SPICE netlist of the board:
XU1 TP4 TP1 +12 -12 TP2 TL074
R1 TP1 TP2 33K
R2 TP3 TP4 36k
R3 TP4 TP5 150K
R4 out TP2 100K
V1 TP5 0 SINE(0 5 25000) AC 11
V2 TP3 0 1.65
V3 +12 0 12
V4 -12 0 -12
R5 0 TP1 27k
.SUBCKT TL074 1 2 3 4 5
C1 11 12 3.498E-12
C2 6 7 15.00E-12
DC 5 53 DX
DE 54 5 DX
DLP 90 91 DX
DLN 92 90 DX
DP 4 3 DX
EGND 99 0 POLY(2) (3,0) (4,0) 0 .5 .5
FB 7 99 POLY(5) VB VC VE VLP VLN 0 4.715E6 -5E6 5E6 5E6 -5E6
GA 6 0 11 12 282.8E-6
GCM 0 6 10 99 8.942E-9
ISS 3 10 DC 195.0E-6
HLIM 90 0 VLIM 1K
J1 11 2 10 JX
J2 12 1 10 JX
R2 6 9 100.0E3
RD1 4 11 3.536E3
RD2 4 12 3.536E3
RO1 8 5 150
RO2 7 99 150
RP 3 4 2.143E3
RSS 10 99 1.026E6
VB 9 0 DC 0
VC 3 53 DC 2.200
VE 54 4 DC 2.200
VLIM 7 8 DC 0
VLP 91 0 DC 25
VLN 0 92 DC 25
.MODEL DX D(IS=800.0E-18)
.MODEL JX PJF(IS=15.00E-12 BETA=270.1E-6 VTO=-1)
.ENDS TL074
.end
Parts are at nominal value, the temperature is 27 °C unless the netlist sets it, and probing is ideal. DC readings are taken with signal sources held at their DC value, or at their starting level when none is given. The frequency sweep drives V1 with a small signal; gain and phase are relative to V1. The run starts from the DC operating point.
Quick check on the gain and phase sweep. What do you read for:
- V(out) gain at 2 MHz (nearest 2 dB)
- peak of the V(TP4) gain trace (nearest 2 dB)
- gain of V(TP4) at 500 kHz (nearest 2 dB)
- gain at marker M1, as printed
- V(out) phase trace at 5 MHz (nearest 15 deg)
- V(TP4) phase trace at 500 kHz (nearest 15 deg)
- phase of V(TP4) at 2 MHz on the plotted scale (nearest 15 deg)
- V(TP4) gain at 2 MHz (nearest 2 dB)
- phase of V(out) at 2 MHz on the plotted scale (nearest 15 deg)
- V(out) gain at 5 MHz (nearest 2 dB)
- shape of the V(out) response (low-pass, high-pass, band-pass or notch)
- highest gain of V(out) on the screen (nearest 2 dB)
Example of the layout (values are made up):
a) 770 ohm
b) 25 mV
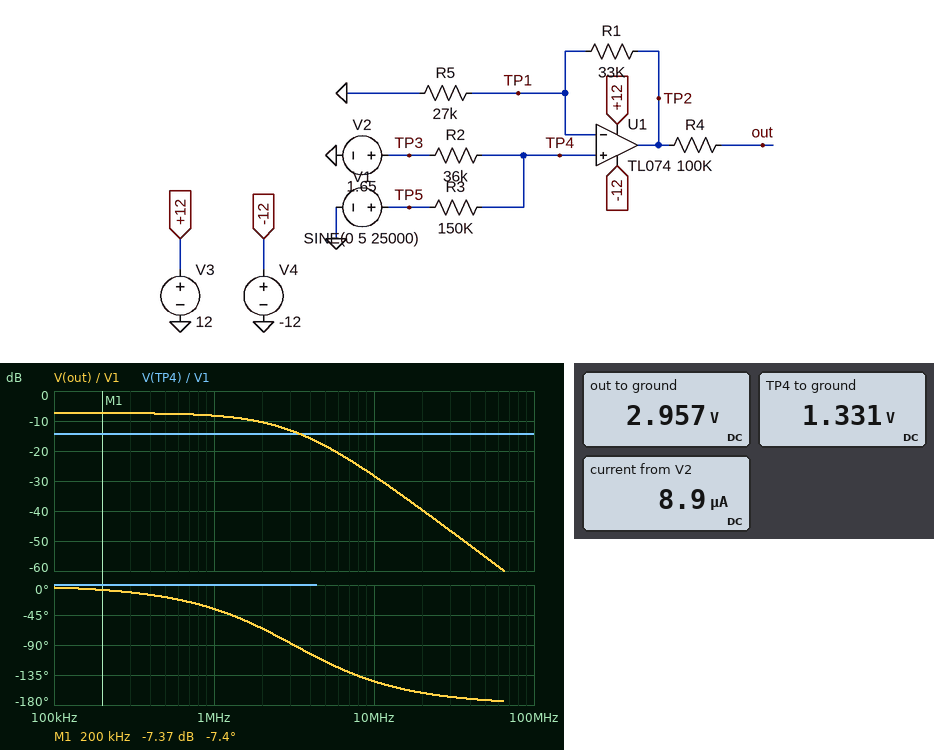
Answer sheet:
a) -10 dB
b) -14 dB
c) -14 dB
d) -7.37 dB
e) -120 deg
f) 0 deg
g) 0 deg
h) -14 dB
i) -60 deg
j) -18 dB
k) low-pass
l) -8 dB
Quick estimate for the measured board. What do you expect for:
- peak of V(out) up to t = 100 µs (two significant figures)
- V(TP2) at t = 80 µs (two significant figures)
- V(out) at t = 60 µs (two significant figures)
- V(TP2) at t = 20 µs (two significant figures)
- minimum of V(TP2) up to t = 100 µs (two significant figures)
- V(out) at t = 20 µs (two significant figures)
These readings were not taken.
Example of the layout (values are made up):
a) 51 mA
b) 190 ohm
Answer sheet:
a) 5.1 V
b) 2.9 V
c) 3.0 V
d) 3.0 V
e) 810 mV
f) 3.0 V
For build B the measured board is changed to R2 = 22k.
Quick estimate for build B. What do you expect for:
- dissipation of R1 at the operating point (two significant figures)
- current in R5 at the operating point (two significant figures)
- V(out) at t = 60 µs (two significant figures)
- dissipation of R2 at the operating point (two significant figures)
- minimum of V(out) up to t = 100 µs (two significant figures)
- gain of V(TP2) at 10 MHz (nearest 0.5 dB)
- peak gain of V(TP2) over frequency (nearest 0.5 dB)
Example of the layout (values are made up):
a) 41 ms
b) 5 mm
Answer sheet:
a) 94 µW
b) 53 µA
c) 3.2 V
d) 2.0 µW
e) 1.8 V
f) -32.0 dB
g) -11.0 dB
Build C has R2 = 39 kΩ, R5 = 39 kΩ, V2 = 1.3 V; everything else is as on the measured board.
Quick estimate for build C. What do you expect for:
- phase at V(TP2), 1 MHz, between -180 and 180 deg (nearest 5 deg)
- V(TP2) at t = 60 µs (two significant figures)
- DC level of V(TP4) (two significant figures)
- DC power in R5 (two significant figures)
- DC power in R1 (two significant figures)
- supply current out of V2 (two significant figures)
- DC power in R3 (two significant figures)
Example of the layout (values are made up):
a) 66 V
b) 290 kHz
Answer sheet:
a) -30 deg
b) 1.9 V
c) 1.0 V
d) 27 µW
e) 23 µW
f) 6.9 µA
g) 7.1 µW
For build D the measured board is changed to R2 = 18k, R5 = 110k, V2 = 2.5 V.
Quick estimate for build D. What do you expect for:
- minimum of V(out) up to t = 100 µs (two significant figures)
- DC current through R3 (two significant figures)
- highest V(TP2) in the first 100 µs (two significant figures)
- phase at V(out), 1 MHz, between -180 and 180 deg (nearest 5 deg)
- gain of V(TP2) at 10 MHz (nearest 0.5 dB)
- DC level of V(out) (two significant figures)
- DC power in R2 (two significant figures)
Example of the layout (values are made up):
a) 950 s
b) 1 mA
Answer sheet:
a) 2.2 V
b) 15 µA
c) 3.6 V
d) -20 deg
e) -33.0 dB
f) 2.9 V
g) 4.0 µW
